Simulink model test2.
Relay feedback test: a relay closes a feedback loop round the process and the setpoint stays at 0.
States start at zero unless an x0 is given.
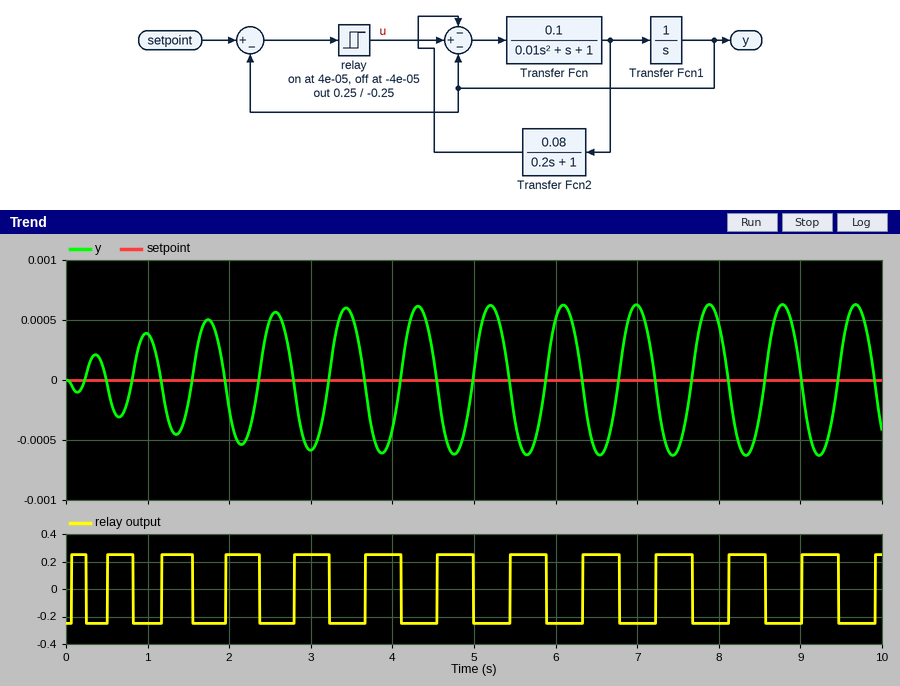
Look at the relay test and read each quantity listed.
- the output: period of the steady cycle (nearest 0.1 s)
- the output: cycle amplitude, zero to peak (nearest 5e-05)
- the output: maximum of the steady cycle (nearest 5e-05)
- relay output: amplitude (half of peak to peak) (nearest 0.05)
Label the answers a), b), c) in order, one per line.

a) 0.9 s
b) 0.00065
c) 0.00065
d) 0.25
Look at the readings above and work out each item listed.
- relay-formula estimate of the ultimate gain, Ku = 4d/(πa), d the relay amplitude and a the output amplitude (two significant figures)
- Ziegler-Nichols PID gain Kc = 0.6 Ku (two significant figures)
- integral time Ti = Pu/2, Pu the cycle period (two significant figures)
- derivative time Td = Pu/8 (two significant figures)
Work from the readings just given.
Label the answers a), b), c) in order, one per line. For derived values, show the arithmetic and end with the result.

a) 4 × 0.25 / (π × 0.00065) = 490
b) 0.6 × 490 = 290
c) 0.9 / 2 = 0.45 s
d) 0.9 / 8 = 0.11 s
